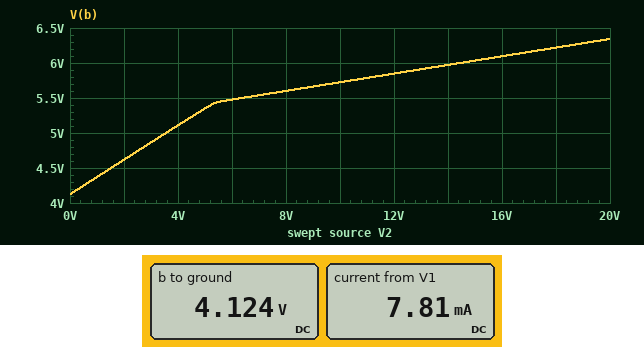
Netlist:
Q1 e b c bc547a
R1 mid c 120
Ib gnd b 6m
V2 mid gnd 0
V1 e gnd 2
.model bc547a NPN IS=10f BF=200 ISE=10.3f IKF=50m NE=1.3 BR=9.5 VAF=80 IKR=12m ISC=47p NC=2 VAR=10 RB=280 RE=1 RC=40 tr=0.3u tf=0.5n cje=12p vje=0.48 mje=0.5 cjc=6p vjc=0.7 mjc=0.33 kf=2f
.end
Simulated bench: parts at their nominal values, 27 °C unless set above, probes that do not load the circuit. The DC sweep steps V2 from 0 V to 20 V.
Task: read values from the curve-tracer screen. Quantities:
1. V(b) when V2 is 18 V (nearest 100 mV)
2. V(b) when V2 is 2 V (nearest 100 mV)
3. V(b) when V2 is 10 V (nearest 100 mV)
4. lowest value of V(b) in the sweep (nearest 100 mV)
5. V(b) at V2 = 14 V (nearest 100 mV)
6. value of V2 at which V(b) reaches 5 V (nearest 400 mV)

6.2 V
4.6 V
5.7 V
4.1 V
6.0 V
3.6 V
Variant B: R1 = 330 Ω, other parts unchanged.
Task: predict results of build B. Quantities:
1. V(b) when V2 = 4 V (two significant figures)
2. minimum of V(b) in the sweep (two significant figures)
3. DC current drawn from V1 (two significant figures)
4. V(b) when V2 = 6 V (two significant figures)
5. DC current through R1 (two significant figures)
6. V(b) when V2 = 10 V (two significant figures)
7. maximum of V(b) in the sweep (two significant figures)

4.9 V
4.4 V
17 µA
5.1 V
6.0 mA
5.5 V
5.9 V
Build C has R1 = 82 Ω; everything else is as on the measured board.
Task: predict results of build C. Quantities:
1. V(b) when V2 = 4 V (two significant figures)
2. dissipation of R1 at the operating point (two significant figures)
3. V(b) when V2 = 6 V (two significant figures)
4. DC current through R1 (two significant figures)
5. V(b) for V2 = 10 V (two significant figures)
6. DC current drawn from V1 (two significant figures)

5.2 V
27 mW
5.5 V
18 mA
5.8 V
12 mA
